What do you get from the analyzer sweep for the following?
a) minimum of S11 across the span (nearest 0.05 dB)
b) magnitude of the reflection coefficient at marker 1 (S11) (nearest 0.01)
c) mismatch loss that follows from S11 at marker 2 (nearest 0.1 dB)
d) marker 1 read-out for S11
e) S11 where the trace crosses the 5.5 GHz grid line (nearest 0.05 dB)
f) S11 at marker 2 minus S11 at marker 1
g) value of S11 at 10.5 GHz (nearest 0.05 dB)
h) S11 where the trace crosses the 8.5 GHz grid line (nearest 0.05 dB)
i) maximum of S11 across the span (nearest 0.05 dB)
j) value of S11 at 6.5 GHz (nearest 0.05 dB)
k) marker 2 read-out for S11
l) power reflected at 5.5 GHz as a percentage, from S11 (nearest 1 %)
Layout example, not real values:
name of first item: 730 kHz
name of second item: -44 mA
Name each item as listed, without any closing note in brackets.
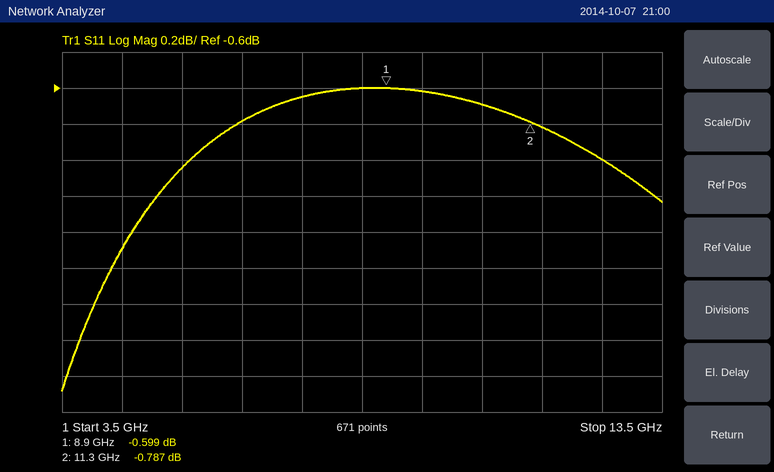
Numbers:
minimum of S11 across the span: -2.30 dB
magnitude of the reflection coefficient at marker 1 (S11): 0.93
mismatch loss that follows from S11 at marker 2: 7.8 dB
marker 1 read-out for S11: -0.599 dB
S11 where the trace crosses the 5.5 GHz grid line: -1.05 dB
S11 at marker 2 minus S11 at marker 1: -0.188 dB
value of S11 at 10.5 GHz: -0.70 dB
S11 where the trace crosses the 8.5 GHz grid line: -0.60 dB
maximum of S11 across the span: -0.60 dB
value of S11 at 6.5 GHz: -0.80 dB
marker 2 read-out for S11: -0.787 dB
power reflected at 5.5 GHz as a percentage, from S11: 79 %
